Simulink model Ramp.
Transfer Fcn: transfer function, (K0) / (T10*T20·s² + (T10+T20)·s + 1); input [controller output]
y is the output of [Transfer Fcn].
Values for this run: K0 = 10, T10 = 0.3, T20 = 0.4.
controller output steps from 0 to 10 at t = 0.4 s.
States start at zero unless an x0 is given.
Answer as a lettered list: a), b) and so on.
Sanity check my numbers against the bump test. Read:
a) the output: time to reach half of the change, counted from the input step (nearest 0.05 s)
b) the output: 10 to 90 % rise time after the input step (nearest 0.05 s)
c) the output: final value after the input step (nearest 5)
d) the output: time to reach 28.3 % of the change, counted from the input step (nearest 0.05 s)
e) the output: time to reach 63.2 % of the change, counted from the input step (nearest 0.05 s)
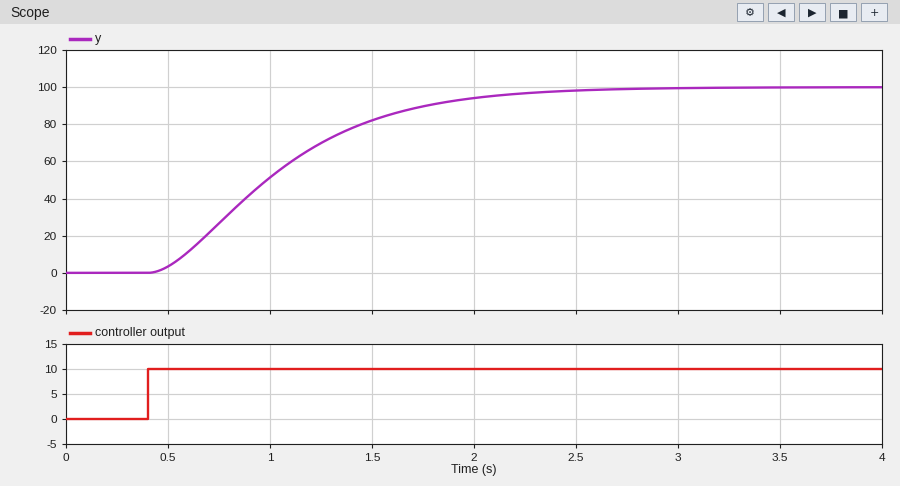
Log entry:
a) 0.60 s
b) 1.20 s
c) 100
d) 0.35 s
e) 0.75 s
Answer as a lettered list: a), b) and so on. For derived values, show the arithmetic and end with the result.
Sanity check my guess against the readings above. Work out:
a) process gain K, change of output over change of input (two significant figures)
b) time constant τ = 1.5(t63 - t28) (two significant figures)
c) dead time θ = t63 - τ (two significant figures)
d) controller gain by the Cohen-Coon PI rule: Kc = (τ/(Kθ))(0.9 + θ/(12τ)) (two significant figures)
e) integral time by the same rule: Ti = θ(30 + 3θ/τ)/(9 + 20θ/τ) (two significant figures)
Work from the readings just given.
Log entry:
a) (100 - 0) / 10 = 10
b) 1.5 × (0.75 - 0.35) = 0.60 s
c) 0.75 - 0.6 = 0.15 s
d) 0.6 / (10 × 0.15) × (0.9 + 0.15 / (12 × 0.6)) = 0.37
e) 0.15 × (30 + 3 × 0.15 / 0.6) / (9 + 20 × 0.15 / 0.6) = 0.33 s
